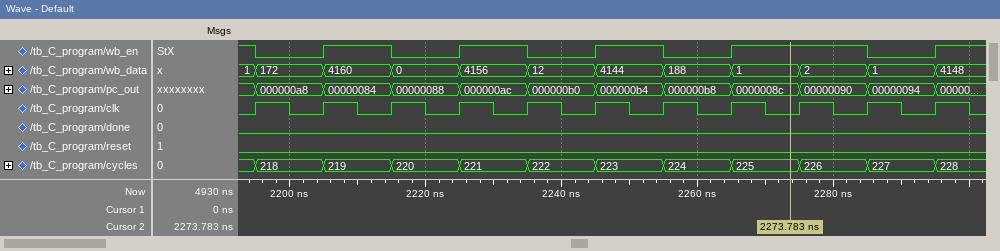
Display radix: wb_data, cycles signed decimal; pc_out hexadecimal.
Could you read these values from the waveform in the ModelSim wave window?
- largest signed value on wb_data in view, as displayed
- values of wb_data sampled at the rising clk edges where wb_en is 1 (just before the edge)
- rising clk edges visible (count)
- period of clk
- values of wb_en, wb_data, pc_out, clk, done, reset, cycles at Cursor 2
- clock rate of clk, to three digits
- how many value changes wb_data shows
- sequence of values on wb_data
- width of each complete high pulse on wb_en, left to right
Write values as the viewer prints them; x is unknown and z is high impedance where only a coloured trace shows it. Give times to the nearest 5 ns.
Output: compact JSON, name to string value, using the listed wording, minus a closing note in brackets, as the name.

{"largest signed value on wb_data in view, as displayed": "4160", "values of wb_data sampled at the rising clk edges where wb_en is 1": "1, 4160, 4156, 4144, 1, 2", "rising clk edges visible": "11", "period of clk": "10 ns", "values of wb_en, wb_data, pc_out, clk, done, reset, cycles at Cursor 2": "wb_en=1, wb_data=1, pc_out=0000008c, clk=0, done=0, reset=0, cycles=225", "clock rate of clk, to three digits": "100 MHz", "how many value changes wb_data shows": "11", "sequence of values on wb_data": "1, 172, 4160, 0, 4156, 12, 4144, 188, 1, 2, 1, 4148", "width of each complete high pulse on wb_en, left to right": "10 ns, 10 ns, 10 ns, 20 ns"}
